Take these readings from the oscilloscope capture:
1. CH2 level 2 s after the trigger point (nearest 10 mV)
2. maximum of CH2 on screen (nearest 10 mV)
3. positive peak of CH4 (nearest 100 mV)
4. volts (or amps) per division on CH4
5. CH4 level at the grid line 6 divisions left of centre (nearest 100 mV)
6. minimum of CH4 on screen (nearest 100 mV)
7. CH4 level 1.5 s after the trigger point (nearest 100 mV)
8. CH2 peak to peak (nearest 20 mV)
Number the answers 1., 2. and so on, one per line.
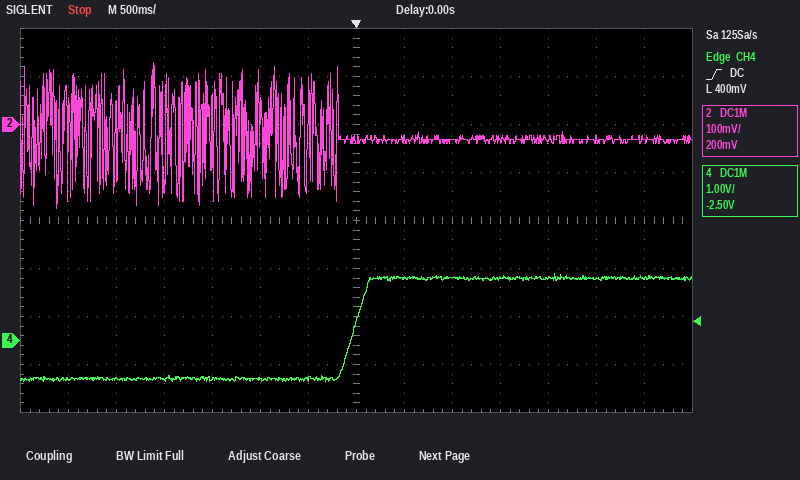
1. -30 mV
2. 130 mV
3. 1.4 V
4. 1 V
5. -800 mV
6. -900 mV
7. 1.3 V
8. 300 mV
